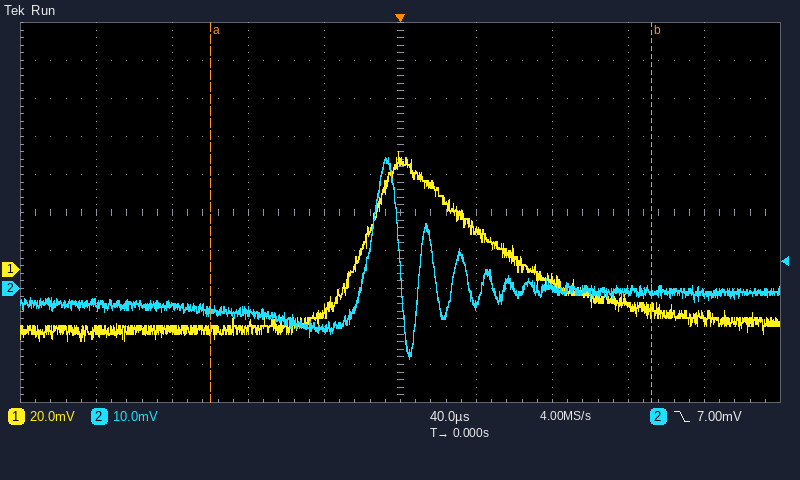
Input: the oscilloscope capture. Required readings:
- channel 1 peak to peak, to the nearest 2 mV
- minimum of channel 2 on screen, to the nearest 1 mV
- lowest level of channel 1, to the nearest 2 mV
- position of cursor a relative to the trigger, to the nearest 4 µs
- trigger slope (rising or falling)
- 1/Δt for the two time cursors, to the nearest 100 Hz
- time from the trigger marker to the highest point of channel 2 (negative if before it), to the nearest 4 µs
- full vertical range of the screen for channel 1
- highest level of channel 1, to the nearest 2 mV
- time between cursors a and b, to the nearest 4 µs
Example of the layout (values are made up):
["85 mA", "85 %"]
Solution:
["100 mV", "-18 mV", "-38 mV", "-100 µs", "falling", "4.3 kHz", "-8 µs", "200 mV", "62 mV", "232 µs"]
